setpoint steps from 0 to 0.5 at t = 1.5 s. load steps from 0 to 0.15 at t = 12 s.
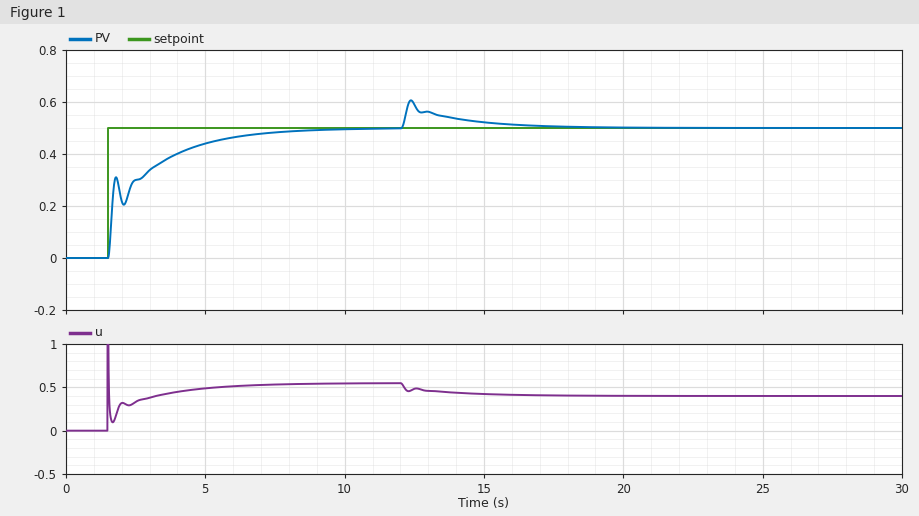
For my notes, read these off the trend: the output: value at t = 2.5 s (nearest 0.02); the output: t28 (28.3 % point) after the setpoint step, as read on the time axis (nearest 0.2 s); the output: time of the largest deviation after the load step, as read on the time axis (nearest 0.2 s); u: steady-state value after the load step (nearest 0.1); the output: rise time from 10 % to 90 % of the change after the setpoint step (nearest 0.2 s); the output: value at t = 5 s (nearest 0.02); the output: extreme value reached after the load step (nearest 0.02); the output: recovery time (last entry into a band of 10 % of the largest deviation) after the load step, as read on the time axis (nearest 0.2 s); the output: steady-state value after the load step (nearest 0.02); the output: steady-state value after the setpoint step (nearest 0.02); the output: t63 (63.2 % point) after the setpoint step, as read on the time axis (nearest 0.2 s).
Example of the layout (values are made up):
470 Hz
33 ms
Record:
0.30
1.6 s
12.4 s
0.4
3.8 s
0.44
0.60
16.4 s
0.50
0.50
2.8 s
